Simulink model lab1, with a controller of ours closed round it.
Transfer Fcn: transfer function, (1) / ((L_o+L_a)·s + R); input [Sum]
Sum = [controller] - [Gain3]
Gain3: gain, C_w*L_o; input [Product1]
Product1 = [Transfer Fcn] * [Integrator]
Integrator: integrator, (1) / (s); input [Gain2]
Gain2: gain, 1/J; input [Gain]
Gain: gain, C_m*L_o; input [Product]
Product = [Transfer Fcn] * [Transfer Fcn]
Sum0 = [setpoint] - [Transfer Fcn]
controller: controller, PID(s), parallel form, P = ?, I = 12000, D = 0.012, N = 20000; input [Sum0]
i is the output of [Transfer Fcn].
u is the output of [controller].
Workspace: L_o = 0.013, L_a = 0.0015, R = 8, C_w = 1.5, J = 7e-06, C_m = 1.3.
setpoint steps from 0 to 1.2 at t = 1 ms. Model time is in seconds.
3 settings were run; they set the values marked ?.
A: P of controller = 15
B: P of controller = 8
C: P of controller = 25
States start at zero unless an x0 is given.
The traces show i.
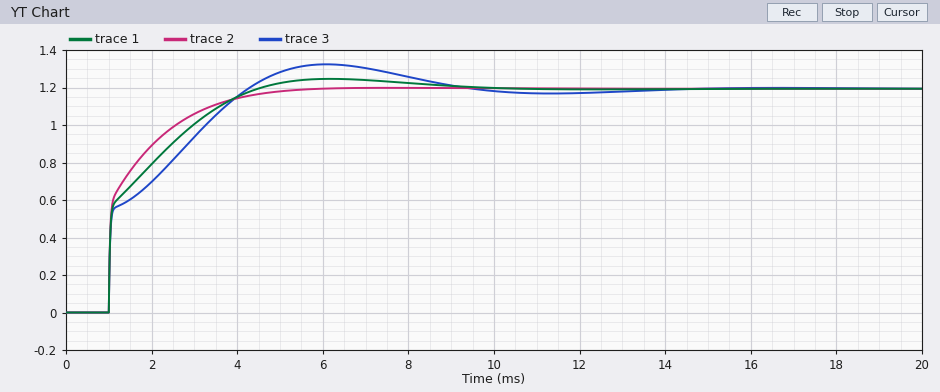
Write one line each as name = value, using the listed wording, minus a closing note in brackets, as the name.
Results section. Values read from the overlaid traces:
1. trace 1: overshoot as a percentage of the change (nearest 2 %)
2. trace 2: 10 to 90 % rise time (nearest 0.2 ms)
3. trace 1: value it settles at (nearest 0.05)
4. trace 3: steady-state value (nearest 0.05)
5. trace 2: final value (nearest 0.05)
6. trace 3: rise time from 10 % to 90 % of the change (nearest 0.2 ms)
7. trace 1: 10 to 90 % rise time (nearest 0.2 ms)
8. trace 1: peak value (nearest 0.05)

trace 1: overshoot as a percentage of the change = 4 %
trace 2: 10 to 90 % rise time = 2.2 ms
trace 1: value it settles at = 1.20
trace 3: steady-state value = 1.20
trace 2: final value = 1.20
trace 3: rise time from 10 % to 90 % of the change = 2.6 ms
trace 1: 10 to 90 % rise time = 2.4 ms
trace 1: peak value = 1.25
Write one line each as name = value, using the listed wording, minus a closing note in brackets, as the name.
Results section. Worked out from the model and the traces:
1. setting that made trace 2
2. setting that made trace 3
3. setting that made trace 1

setting that made trace 2 = C
setting that made trace 3 = B
setting that made trace 1 = A
